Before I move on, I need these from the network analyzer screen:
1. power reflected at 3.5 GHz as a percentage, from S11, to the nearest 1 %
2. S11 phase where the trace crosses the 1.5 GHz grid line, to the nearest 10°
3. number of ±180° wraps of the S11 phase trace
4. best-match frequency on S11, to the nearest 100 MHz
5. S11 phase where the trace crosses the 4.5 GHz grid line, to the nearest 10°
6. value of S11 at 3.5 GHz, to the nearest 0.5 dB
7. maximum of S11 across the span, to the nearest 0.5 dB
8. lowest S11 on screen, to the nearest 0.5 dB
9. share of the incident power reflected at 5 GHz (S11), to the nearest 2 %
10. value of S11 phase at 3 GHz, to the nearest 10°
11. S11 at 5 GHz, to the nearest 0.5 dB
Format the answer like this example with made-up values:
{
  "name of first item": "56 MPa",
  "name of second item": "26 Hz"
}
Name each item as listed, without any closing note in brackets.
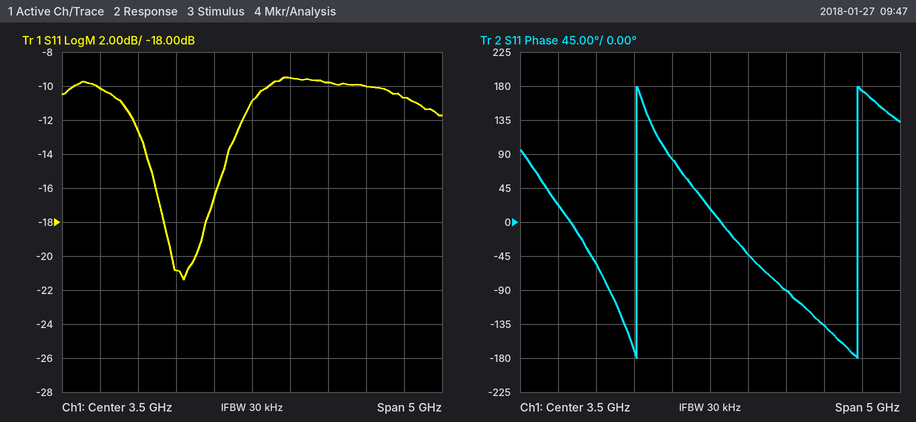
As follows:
{
  "power reflected at 3.5 GHz as a percentage, from S11, to the nearest 1 %": "8 %",
  "S11 phase where the trace crosses the 1.5 GHz grid line, to the nearest 10°": "20°",
  "number of ±180° wraps of the S11 phase trace": "2",
  "best-match frequency on S11, to the nearest 100 MHz": "2.6 GHz",
  "S11 phase where the trace crosses the 4.5 GHz grid line, to the nearest 10°": "-90°",
  "value of S11 at 3.5 GHz, to the nearest 0.5 dB": "-11.0 dB",
  "maximum of S11 across the span, to the nearest 0.5 dB": "-9.5 dB",
  "lowest S11 on screen, to the nearest 0.5 dB": "-21.5 dB",
  "share of the incident power reflected at 5 GHz (S11), to the nearest 2 %": "10 %",
  "value of S11 phase at 3 GHz, to the nearest 10°": "80°",
  "S11 at 5 GHz, to the nearest 0.5 dB": "-10.0 dB"
}
